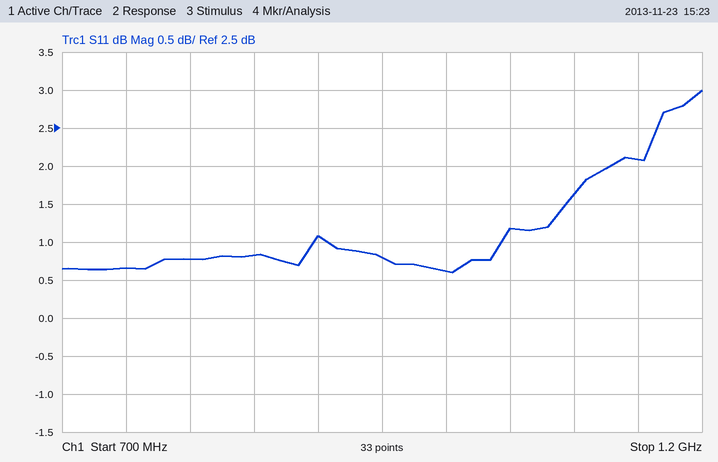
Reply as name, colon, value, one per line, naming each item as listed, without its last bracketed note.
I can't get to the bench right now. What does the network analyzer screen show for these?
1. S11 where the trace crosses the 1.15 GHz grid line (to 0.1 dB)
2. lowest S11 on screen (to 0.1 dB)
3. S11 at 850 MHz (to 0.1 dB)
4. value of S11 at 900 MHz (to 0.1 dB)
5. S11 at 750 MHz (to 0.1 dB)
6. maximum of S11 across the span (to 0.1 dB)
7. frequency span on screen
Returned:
S11 where the trace crosses the 1.15 GHz grid line: 2.1 dB
lowest S11 on screen: 0.6 dB
S11 at 850 MHz: 0.8 dB
value of S11 at 900 MHz: 1.1 dB
S11 at 750 MHz: 0.7 dB
maximum of S11 across the span: 3.0 dB
frequency span on screen: 500 MHz
